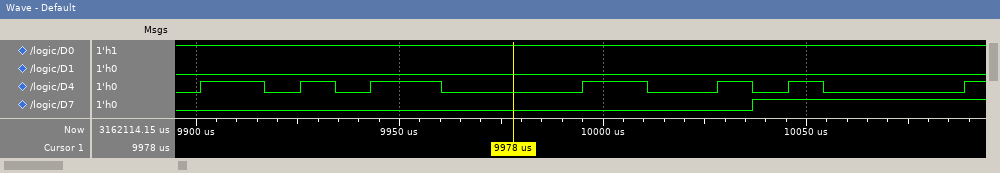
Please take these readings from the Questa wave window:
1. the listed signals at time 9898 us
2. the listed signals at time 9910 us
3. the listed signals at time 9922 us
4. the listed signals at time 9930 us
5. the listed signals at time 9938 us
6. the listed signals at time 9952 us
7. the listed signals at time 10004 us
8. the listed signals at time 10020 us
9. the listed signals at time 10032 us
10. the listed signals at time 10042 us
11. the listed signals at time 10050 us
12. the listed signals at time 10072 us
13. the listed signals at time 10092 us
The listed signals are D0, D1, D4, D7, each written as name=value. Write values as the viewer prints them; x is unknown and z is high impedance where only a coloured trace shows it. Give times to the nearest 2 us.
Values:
D0=1, D1=0, D4=0, D7=0
D0=1, D1=0, D4=1, D7=0
D0=1, D1=0, D4=0, D7=0
D0=1, D1=0, D4=1, D7=0
D0=1, D1=0, D4=0, D7=0
D0=1, D1=0, D4=1, D7=0
D0=1, D1=0, D4=1, D7=0
D0=1, D1=0, D4=0, D7=0
D0=1, D1=0, D4=1, D7=0
D0=1, D1=0, D4=0, D7=1
D0=1, D1=0, D4=1, D7=1
D0=1, D1=0, D4=0, D7=1
D0=1, D1=0, D4=1, D7=1
